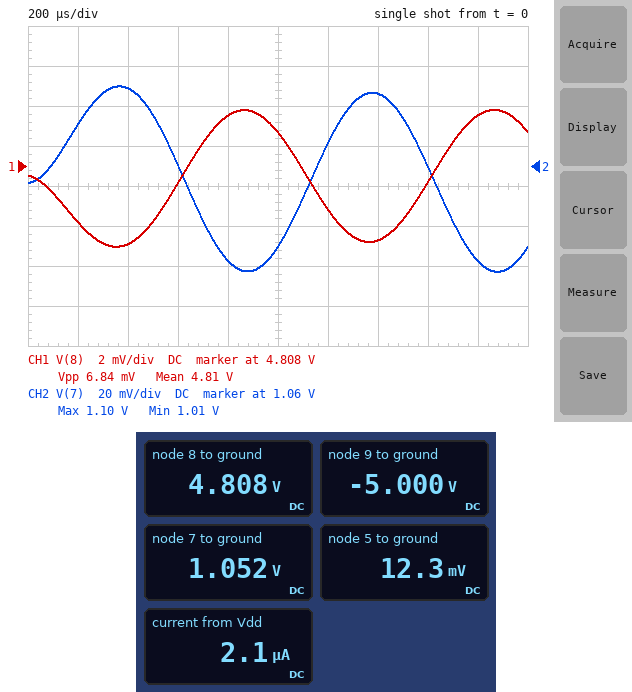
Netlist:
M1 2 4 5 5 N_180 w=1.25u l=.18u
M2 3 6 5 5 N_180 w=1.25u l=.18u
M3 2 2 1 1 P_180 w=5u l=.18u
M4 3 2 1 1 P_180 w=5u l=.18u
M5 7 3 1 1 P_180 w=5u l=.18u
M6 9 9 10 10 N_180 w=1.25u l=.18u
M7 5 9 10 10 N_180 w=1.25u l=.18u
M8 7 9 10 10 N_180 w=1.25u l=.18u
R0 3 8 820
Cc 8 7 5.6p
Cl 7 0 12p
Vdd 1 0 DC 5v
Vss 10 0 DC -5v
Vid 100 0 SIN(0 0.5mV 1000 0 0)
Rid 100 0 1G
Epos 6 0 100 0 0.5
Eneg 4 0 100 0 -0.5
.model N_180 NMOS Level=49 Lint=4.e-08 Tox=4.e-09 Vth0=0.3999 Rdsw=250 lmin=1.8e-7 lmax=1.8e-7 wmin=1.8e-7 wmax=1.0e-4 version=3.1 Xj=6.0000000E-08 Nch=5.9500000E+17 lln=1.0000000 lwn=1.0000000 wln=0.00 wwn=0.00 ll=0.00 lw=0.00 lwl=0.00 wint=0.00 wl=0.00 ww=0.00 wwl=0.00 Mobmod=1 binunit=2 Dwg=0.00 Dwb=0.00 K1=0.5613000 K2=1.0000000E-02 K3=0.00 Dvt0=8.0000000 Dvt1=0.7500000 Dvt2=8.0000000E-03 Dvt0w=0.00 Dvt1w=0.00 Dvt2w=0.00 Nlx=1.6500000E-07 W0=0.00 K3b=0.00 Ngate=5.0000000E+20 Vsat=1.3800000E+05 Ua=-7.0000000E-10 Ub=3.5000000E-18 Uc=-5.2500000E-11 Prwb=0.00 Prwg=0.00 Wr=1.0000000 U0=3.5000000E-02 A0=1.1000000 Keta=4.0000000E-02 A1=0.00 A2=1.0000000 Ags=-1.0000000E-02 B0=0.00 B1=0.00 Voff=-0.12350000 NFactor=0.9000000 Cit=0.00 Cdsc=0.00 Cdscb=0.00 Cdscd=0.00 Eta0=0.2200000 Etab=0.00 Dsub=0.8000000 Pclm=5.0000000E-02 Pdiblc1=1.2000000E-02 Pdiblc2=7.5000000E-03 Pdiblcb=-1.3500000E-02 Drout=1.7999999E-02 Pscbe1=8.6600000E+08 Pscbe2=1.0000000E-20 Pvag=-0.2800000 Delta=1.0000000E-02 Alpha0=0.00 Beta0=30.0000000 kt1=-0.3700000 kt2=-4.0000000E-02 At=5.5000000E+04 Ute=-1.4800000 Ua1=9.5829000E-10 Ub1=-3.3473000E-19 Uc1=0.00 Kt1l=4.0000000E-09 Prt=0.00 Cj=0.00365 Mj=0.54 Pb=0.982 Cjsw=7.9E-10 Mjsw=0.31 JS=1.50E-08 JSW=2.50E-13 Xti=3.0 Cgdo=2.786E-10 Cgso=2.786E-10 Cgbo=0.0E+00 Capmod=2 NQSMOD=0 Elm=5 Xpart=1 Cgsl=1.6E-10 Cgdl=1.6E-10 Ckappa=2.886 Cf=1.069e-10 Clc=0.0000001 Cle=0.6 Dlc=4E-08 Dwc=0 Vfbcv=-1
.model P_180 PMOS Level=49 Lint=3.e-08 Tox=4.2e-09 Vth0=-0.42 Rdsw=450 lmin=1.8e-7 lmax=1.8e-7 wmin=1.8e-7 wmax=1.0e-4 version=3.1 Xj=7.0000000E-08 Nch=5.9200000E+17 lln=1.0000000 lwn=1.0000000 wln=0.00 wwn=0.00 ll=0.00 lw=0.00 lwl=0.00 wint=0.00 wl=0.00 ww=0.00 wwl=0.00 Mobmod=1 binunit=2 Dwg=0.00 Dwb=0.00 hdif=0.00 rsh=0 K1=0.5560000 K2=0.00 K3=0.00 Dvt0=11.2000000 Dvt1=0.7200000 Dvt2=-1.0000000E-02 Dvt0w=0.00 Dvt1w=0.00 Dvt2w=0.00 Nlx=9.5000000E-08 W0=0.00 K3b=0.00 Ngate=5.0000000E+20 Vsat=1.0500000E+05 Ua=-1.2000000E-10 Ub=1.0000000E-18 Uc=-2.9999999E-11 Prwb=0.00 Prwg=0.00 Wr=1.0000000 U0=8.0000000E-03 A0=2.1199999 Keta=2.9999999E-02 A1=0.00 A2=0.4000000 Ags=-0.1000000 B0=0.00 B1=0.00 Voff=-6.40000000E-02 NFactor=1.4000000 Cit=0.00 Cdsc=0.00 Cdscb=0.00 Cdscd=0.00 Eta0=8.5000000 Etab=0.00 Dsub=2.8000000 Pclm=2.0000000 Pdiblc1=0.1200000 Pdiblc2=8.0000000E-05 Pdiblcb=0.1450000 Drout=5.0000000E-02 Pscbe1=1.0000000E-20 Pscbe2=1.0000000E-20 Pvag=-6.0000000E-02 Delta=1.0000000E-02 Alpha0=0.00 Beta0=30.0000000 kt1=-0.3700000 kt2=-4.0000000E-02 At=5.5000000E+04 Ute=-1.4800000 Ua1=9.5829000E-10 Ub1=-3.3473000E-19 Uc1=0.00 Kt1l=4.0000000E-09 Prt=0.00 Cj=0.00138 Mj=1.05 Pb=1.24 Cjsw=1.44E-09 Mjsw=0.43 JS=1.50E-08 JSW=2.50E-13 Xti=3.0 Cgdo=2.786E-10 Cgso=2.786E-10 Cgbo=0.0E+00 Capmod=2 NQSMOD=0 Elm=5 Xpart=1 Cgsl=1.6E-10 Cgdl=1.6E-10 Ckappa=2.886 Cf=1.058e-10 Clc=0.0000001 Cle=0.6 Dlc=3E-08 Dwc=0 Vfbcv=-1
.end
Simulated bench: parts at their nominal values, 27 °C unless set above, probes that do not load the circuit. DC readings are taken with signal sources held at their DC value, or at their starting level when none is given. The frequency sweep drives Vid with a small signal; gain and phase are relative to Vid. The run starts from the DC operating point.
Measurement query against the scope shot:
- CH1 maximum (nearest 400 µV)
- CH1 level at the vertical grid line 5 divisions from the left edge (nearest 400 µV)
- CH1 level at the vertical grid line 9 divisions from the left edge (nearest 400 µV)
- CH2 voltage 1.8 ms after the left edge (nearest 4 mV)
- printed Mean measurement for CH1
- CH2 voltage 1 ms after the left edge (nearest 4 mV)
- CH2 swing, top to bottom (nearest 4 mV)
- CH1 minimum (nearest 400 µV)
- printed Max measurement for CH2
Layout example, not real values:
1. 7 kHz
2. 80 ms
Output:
1. 4.8108 V
2. 4.8096 V
3. 4.8104 V
4. 1.012 V
5. 4.81 V
6. 1.020 V
7. 92 mV
8. 4.8040 V
9. 1.10 V
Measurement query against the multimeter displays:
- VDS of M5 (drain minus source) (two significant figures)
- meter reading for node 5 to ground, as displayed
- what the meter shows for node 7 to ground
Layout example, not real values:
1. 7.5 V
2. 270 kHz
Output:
1. -3.9 V
2. 12.3 mV
3. 1.052 V
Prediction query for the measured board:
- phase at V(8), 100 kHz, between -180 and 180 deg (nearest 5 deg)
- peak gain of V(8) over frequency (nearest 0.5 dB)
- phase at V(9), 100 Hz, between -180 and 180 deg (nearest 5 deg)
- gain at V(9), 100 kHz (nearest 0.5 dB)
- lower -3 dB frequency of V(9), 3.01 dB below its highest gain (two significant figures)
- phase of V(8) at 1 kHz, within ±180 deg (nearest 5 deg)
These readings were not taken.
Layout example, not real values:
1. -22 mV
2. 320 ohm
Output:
1. 140 deg
2. 19.5 dB
3. 85 deg
4. -18.0 dB
5. 920 Hz
6. 140 deg
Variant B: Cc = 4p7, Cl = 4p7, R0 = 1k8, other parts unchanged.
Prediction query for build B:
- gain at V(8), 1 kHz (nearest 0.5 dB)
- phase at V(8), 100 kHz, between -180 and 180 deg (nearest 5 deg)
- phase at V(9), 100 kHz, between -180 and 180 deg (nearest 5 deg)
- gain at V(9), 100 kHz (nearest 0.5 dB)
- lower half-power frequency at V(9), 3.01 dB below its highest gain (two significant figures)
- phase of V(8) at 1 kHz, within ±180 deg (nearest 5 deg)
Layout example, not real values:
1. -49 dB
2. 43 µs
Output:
1. 17.0 dB
2. 130 deg
3. -80 deg
4. -16.5 dB
5. 1.1 kHz
6. 145 deg
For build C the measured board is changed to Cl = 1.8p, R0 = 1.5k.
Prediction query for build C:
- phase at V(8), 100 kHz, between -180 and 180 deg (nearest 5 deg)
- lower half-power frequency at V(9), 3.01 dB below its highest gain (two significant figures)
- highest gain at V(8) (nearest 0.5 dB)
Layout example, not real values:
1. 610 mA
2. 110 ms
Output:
1. 125 deg
2. 940 Hz
3. 19.5 dB
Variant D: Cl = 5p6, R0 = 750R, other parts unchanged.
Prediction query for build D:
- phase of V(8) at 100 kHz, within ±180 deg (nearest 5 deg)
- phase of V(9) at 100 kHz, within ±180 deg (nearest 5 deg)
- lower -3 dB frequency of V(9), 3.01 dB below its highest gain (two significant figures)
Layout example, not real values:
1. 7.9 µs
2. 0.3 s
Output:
1. 135 deg
2. -80 deg
3. 930 Hz
